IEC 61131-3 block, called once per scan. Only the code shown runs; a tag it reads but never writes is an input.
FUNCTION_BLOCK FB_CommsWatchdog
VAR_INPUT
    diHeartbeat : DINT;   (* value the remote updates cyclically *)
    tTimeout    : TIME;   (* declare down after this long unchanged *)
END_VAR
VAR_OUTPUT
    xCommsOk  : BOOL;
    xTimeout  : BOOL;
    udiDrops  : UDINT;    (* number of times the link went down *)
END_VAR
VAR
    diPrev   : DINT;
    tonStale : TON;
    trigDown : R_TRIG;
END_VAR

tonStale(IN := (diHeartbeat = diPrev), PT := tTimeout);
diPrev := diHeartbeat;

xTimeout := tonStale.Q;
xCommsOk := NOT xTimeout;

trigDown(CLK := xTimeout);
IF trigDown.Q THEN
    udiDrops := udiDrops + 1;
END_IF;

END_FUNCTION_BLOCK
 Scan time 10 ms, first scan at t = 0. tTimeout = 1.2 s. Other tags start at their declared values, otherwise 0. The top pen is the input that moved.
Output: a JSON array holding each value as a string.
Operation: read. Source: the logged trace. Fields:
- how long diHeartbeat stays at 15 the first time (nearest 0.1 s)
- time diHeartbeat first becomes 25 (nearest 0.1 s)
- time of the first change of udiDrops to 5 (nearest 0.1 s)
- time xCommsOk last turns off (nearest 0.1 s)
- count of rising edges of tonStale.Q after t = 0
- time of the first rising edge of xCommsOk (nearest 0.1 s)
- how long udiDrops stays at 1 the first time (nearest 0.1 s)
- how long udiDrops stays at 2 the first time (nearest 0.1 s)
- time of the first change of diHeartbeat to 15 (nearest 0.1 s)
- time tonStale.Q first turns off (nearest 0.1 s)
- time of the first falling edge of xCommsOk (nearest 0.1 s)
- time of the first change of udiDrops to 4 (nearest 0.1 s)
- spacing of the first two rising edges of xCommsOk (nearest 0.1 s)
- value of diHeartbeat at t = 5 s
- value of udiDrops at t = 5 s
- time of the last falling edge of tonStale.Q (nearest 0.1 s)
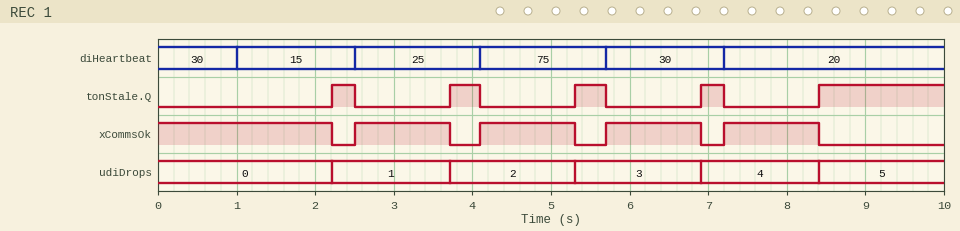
["1.5 s", "2.5 s", "8.4 s", "8.4 s", "5", "2.5 s", "1.5 s", "1.6 s", "1.0 s", "2.5 s", "2.2 s", "6.9 s", "1.6 s", "75", "2", "7.2 s"]
